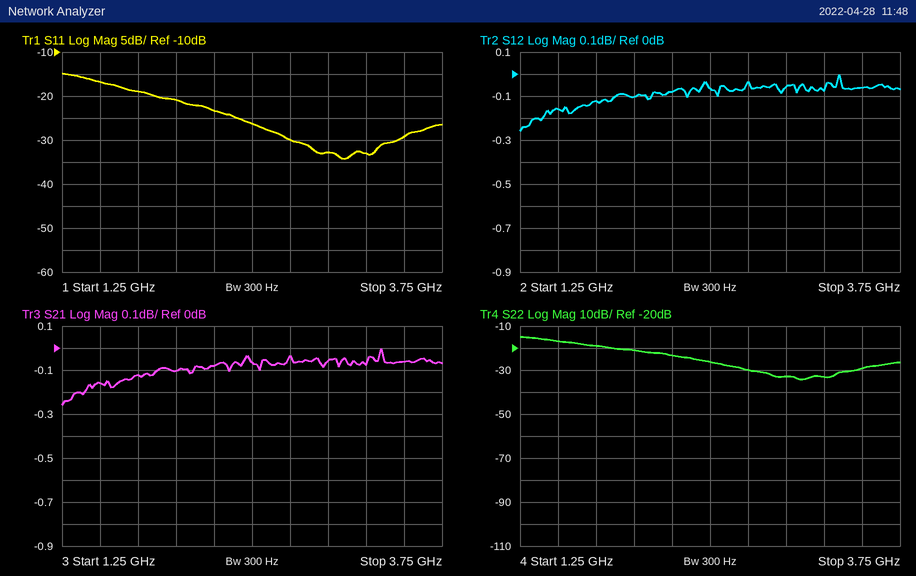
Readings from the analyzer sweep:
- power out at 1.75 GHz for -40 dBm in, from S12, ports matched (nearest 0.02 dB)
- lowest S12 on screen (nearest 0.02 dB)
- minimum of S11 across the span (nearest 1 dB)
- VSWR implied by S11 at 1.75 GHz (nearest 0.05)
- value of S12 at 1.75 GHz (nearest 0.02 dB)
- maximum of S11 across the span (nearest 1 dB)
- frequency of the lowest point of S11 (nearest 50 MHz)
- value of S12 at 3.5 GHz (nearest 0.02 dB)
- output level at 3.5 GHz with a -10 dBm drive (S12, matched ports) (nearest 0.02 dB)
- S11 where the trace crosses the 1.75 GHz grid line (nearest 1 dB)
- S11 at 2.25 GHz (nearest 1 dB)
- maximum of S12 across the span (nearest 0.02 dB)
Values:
-40.12 dBm
-0.26 dB
-34 dB
1.25
-0.12 dB
-15 dB
3.10 GHz
-0.06 dB
-10.06 dBm
-19 dB
-23 dB
0.00 dB
